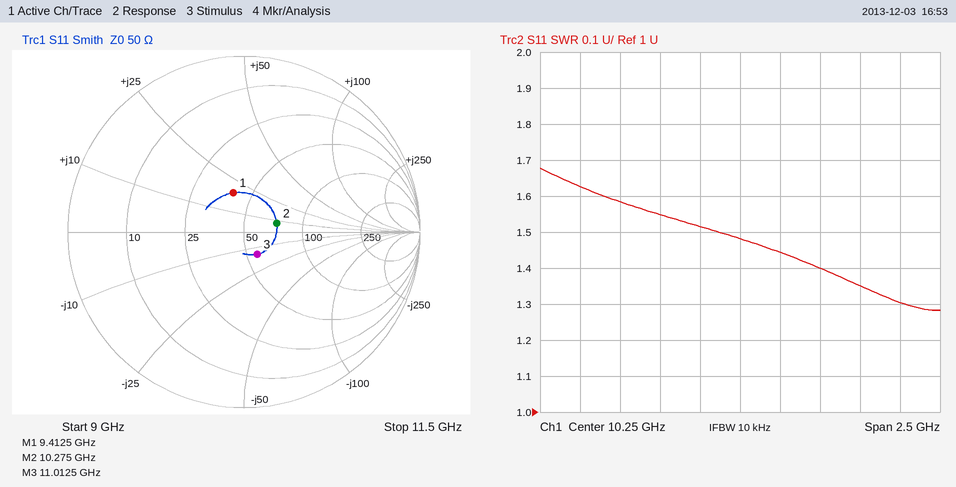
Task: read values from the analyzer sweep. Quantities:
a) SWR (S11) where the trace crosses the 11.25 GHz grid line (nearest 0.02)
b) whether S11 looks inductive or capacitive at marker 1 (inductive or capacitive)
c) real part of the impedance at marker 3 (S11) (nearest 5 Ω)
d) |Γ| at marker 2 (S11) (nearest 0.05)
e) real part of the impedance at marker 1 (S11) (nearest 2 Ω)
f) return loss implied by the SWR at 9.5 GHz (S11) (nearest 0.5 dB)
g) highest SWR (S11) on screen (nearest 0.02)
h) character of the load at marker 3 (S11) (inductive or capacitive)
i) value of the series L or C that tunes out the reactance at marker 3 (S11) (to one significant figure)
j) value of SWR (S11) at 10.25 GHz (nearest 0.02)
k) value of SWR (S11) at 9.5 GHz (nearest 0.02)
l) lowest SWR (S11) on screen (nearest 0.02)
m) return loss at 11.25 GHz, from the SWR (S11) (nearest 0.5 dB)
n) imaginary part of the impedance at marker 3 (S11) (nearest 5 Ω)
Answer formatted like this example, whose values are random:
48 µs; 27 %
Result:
1.30; inductive; 55 Ω; 0.20; 40 Ω; 13.0 dB; 1.68; capacitive; 200 pH; 1.48; 1.58; 1.28; 17.5 dB; -15 Ω
